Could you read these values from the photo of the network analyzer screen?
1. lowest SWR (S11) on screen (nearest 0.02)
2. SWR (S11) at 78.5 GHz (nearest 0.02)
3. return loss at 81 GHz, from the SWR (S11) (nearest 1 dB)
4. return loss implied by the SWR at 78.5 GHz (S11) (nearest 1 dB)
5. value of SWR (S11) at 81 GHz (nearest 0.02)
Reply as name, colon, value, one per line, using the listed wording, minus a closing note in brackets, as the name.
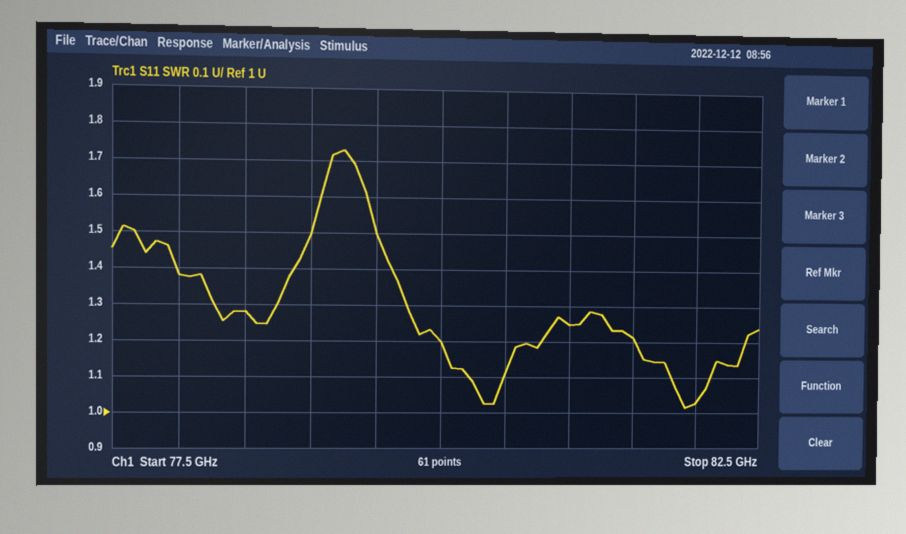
lowest SWR (S11) on screen: 1.02
SWR (S11) at 78.5 GHz: 1.28
return loss at 81 GHz, from the SWR (S11): 19 dB
return loss implied by the SWR at 78.5 GHz (S11): 18 dB
value of SWR (S11) at 81 GHz: 1.24
